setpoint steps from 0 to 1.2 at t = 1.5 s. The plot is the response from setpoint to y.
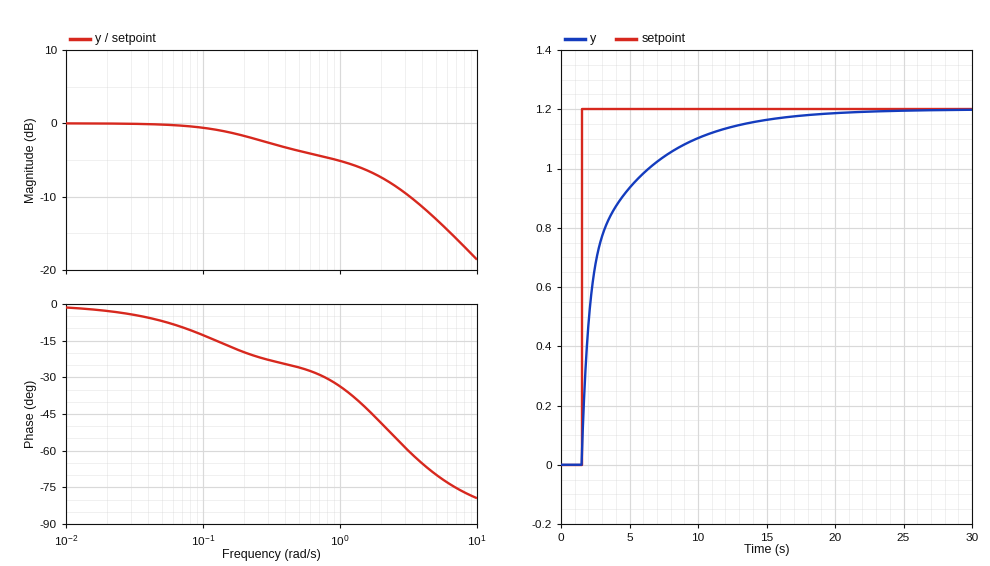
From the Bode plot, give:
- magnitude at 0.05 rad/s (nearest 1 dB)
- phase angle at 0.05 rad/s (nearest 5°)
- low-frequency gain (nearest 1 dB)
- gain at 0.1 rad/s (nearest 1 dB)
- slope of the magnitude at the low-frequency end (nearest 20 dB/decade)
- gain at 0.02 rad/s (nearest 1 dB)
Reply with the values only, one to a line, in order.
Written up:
0 dB
-5°
0 dB
-1 dB
0 dB/decade
0 dB
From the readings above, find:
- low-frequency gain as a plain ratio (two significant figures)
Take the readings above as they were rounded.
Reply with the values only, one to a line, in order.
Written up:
1.0
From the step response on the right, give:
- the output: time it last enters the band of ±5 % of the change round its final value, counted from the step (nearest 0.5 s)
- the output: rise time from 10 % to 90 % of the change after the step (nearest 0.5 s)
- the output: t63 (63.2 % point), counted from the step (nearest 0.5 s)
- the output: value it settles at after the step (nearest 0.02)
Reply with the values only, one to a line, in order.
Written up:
11.0 s
7.5 s
1.5 s
1.20
